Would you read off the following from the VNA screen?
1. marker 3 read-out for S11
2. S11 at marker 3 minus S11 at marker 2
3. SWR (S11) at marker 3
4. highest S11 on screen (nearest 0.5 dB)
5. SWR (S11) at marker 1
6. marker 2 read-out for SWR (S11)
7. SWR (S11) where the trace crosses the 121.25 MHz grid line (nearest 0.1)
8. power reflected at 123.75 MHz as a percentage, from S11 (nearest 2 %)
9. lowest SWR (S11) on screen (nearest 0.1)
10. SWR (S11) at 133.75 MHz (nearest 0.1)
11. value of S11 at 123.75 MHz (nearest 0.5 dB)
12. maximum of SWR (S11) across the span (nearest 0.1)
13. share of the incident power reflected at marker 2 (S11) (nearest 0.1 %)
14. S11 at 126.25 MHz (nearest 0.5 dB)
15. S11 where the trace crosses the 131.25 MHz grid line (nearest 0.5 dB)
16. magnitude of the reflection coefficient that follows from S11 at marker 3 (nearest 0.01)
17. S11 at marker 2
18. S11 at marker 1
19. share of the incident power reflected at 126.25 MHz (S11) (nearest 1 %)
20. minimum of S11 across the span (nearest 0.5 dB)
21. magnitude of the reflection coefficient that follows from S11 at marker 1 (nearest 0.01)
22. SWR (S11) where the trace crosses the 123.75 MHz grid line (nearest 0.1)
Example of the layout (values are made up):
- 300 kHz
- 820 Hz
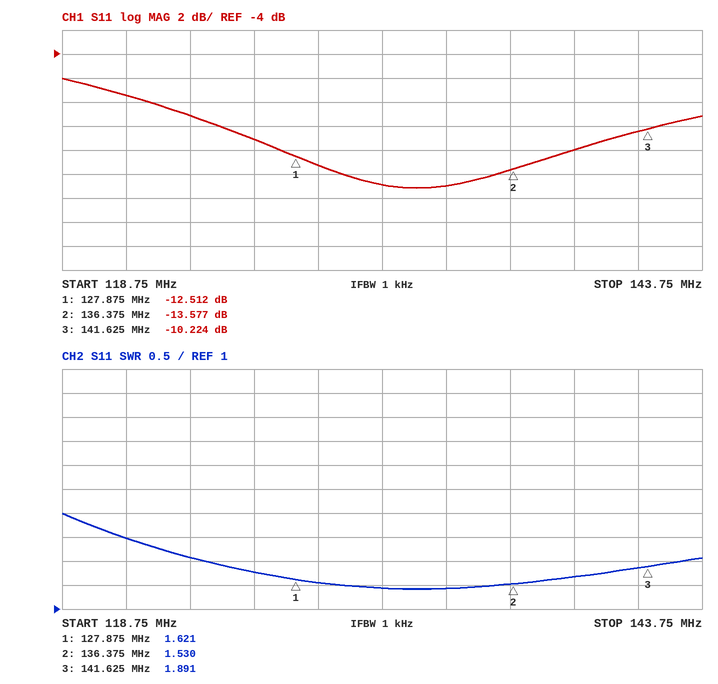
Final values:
- -10.224 dB
- 3.353 dB
- 1.891
- -6.0 dB
- 1.621
- 1.530
- 2.5
- 12 %
- 1.4
- 1.4
- -9.0 dB
- 3.0
- 4.4 %
- -11.0 dB
- -15.0 dB
- 0.31
- -13.577 dB
- -12.512 dB
- 8 %
- -15.0 dB
- 0.24
- 2.1
